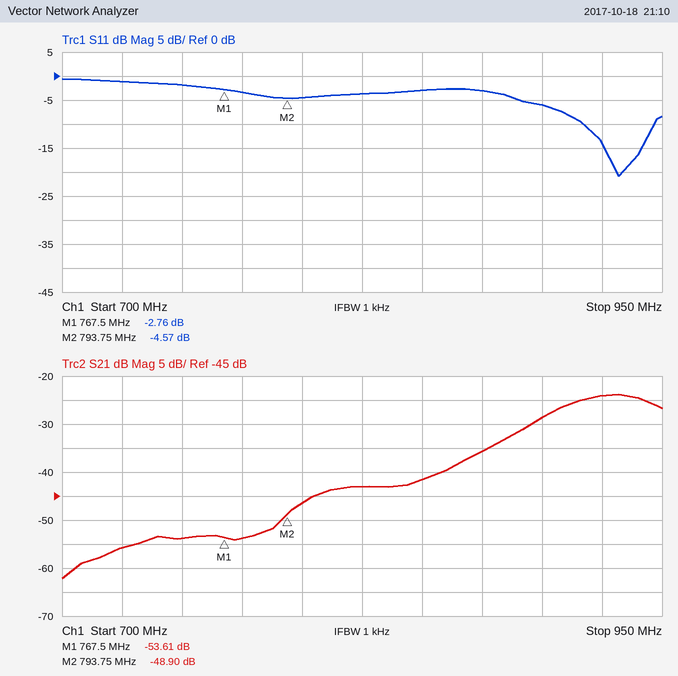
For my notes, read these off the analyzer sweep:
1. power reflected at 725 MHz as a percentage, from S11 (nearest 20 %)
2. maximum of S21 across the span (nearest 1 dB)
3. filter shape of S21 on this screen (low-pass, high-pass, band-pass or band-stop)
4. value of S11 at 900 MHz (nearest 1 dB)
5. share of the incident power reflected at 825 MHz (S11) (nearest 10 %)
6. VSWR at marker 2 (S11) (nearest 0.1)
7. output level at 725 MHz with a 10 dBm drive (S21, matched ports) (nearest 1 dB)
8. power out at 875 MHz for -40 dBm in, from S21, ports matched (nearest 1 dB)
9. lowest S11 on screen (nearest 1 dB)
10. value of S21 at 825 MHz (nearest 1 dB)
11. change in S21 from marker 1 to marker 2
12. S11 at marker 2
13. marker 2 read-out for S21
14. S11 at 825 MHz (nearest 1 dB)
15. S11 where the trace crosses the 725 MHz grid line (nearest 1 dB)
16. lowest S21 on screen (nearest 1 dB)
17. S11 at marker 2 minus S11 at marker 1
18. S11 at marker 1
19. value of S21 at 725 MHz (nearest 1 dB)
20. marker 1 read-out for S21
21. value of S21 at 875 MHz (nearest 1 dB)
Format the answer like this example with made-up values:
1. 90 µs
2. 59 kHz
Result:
1. 80 %
2. -24 dB
3. high-pass
4. -6 dB
5. 40 %
6. 3.9
7. -46 dBm
8. -76 dBm
9. -21 dB
10. -43 dB
11. 4.71 dB
12. -4.57 dB
13. -48.90 dB
14. -4 dB
15. -1 dB
16. -62 dB
17. -1.81 dB
18. -2.76 dB
19. -56 dB
20. -53.61 dB
21. -36 dB
